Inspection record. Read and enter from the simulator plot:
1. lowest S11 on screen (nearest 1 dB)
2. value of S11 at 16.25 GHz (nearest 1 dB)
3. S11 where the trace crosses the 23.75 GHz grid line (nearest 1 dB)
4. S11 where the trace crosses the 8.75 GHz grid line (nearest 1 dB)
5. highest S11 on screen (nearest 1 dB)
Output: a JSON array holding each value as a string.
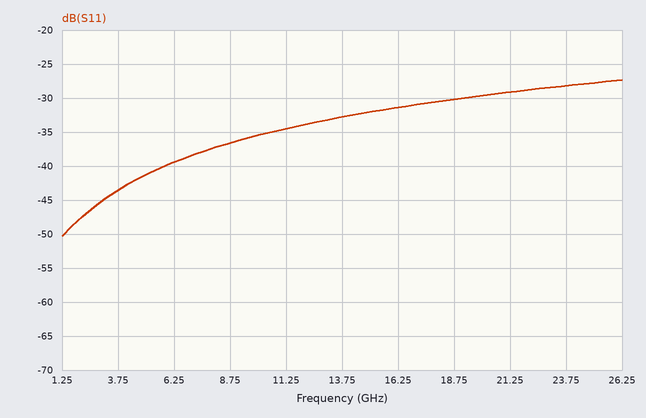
["-50 dB", "-31 dB", "-28 dB", "-37 dB", "-27 dB"]
